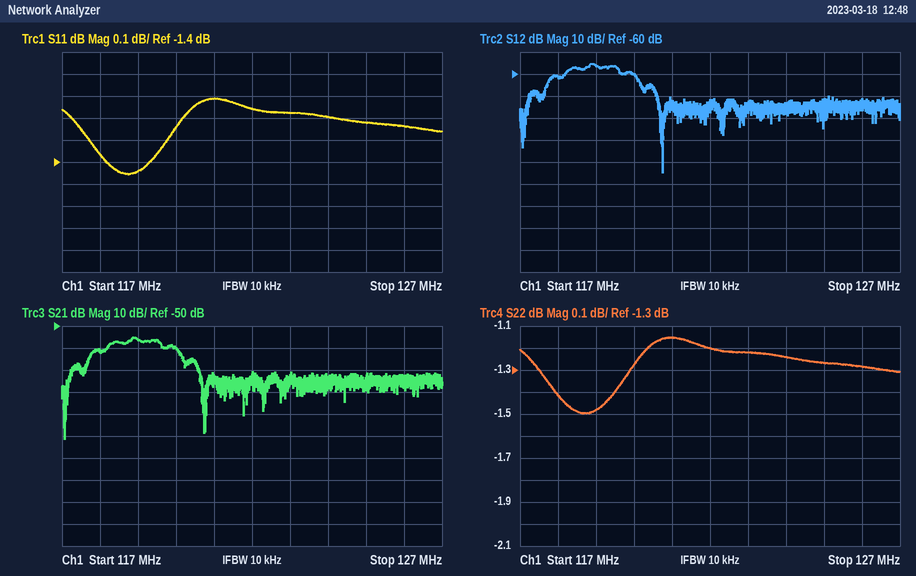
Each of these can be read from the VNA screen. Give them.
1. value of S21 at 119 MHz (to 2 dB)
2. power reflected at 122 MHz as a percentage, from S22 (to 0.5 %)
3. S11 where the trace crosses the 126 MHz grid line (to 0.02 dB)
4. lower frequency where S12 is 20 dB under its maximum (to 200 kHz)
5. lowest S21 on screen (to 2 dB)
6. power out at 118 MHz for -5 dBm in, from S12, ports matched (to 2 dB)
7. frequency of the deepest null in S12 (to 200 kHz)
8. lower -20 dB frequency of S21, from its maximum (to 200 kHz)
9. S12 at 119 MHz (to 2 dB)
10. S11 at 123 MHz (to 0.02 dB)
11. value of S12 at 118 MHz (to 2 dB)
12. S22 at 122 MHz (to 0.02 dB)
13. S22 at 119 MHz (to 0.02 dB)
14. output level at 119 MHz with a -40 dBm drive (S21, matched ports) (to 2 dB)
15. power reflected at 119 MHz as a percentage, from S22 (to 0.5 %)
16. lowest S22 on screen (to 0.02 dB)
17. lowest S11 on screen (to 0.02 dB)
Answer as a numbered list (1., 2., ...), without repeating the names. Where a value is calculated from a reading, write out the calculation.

1. -56 dB
2. 10^(-1.2/10) ≈ 75.9 %, so 76.0 % to the nearest 0.5 %
3. -1.24 dB
4. 117.2 MHz
5. -102 dB
6. -5 dBm + (-62 dB) = -66 dBm
7. 120.8 MHz
8. 117.2 MHz
9. -56 dB
10. -1.18 dB
11. -62 dB
12. -1.20 dB
13. -1.48 dB
14. -40 dBm + (-56 dB) = -96 dBm
15. 10^(-1.48/10) ≈ 71.1 %, so 71.0 % to the nearest 0.5 %
16. -1.50 dB
17. -1.46 dB
